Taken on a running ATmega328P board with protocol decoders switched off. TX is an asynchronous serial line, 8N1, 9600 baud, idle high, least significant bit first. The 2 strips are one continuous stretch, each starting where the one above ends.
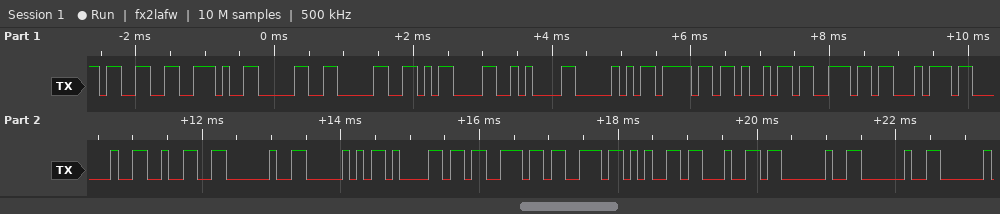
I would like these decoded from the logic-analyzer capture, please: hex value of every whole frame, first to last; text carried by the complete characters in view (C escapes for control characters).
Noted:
33 2E 30 30 0D 0A 50 6F 69 6E 74 20 32 20 50 61 73 73 65 64 20 20
"3.00\r\nPoint 2 Passed  "
